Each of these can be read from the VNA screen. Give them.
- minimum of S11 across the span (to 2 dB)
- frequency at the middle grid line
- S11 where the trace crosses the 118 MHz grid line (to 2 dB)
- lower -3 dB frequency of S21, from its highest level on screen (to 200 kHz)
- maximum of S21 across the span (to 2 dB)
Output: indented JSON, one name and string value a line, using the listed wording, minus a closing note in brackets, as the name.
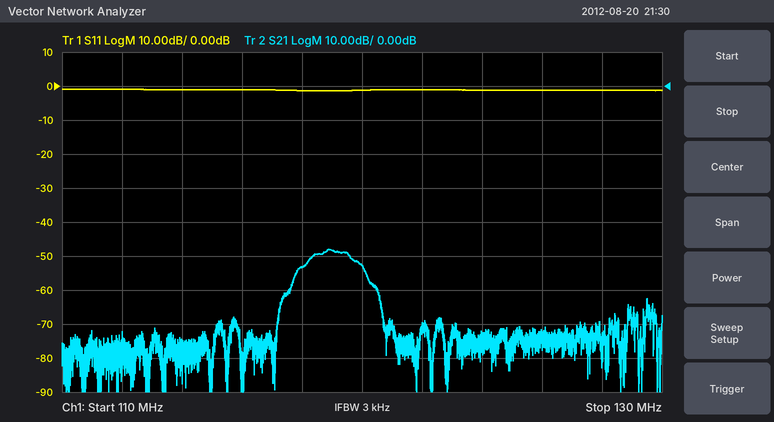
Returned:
{
  "minimum of S11 across the span": "-2 dB",
  "frequency at the middle grid line": "120 MHz",
  "S11 where the trace crosses the 118 MHz grid line": "-2 dB",
  "lower -3 dB frequency of S21, from its highest level on screen": "118.2 MHz",
  "maximum of S21 across the span": "-48 dB"
}
